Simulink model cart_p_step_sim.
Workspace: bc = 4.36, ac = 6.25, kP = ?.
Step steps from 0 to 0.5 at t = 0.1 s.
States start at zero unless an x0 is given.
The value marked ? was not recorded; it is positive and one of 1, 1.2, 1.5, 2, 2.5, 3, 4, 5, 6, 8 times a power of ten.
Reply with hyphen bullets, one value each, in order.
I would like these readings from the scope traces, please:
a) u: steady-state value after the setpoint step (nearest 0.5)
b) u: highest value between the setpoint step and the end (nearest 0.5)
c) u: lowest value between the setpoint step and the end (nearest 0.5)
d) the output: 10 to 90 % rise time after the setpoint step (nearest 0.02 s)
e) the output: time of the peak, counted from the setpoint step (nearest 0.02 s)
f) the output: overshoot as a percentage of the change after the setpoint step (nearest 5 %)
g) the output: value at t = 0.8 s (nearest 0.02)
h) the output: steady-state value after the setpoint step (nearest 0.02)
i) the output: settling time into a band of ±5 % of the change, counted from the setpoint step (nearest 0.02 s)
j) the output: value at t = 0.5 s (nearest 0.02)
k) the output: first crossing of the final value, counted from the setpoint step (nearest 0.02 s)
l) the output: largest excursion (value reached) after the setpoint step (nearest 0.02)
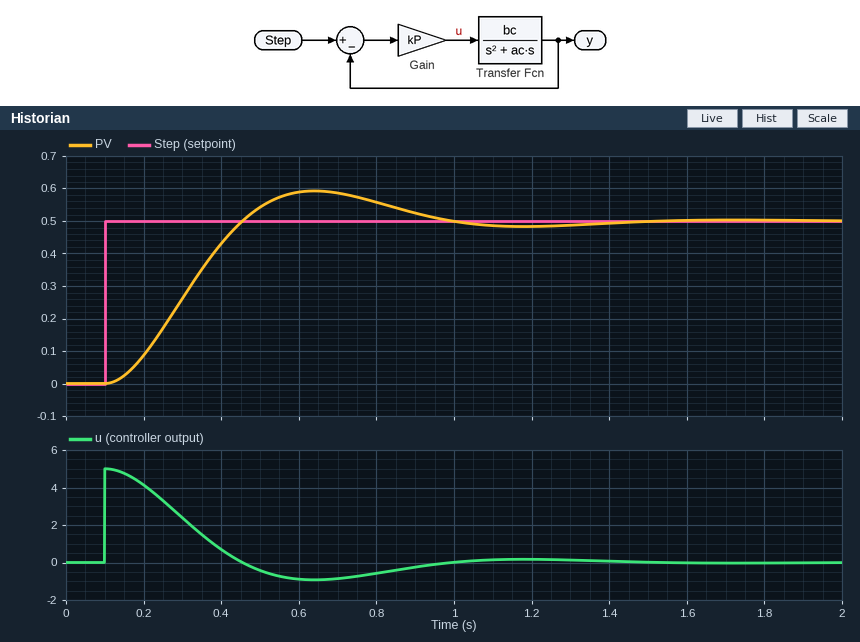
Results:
- 0.0
- 5.0
- -1.0
- 0.24 s
- 0.54 s
- 20 %
- 0.56
- 0.50
- 0.80 s
- 0.54
- 0.36 s
- 0.60
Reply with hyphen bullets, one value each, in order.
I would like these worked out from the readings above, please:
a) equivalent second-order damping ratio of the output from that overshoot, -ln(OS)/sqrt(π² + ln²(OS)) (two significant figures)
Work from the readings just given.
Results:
- 0.46
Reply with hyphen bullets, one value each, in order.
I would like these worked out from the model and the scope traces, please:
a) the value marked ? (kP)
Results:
- 10
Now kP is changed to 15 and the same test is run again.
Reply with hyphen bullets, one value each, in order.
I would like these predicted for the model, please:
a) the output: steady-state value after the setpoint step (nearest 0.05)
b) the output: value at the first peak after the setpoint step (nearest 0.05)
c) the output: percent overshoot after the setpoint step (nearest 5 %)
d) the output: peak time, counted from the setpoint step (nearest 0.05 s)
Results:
- 0.50
- 0.65
- 25 %
- 0.40 s
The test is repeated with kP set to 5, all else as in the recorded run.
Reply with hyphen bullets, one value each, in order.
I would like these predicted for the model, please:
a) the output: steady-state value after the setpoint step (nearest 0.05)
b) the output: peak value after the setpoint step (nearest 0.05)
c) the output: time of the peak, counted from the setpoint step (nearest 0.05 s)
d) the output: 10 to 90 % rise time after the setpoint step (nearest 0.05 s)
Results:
- 0.50
- 0.55
- 0.90 s
- 0.45 s
